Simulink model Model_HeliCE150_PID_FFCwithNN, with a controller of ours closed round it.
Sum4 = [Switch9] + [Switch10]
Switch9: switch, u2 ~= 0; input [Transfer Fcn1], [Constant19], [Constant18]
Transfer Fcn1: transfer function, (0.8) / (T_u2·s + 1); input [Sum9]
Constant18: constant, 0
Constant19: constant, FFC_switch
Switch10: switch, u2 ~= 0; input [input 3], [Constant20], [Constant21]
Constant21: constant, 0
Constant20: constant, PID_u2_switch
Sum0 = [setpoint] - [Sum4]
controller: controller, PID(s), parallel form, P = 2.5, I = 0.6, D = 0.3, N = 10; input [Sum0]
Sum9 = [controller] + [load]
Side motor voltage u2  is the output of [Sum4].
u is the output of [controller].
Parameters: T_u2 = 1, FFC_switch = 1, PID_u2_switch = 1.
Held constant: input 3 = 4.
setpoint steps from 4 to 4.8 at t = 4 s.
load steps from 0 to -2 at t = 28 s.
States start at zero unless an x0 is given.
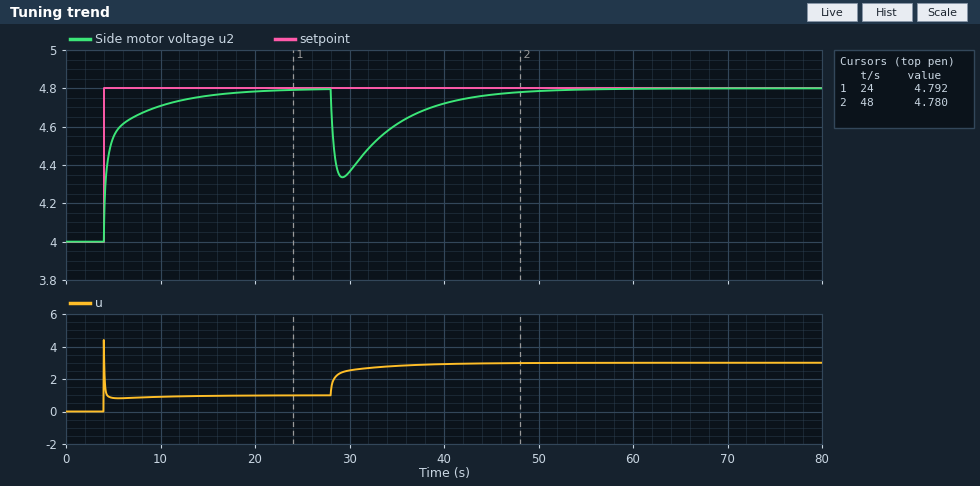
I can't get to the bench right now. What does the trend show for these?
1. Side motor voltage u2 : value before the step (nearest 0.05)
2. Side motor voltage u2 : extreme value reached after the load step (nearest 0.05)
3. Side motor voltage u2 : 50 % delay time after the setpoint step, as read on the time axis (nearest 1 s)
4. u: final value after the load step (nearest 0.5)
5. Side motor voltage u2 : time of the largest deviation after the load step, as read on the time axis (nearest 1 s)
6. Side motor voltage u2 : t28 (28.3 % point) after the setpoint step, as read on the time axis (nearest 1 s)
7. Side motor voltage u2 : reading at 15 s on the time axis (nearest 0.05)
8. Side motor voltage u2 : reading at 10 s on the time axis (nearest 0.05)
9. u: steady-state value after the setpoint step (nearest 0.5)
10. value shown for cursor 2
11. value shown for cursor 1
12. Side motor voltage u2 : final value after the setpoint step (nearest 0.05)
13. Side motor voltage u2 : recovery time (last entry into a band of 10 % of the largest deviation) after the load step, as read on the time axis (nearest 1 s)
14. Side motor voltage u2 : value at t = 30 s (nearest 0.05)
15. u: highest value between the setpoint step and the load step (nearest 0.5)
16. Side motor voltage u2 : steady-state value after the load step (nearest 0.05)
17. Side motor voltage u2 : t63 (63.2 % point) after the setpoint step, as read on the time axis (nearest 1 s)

4.00
4.35
4 s
3.0
29 s
4 s
4.75
4.70
1.0
4.780
4.792
4.80
43 s
4.35
4.5
4.80
5 s
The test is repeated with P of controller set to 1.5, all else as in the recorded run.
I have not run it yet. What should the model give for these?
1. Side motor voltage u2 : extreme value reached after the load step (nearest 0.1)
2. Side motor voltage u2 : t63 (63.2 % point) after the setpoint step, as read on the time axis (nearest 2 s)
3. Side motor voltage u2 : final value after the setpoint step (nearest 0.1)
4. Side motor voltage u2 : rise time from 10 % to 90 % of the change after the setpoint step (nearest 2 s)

4.2
6 s
4.8
6 s
